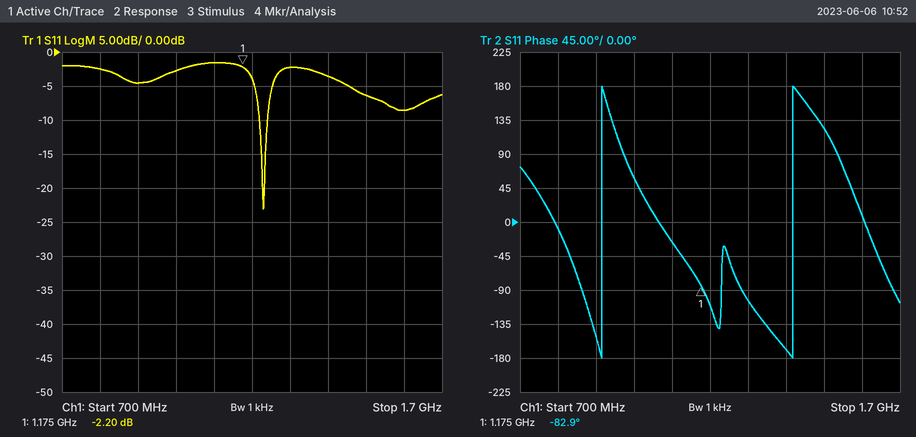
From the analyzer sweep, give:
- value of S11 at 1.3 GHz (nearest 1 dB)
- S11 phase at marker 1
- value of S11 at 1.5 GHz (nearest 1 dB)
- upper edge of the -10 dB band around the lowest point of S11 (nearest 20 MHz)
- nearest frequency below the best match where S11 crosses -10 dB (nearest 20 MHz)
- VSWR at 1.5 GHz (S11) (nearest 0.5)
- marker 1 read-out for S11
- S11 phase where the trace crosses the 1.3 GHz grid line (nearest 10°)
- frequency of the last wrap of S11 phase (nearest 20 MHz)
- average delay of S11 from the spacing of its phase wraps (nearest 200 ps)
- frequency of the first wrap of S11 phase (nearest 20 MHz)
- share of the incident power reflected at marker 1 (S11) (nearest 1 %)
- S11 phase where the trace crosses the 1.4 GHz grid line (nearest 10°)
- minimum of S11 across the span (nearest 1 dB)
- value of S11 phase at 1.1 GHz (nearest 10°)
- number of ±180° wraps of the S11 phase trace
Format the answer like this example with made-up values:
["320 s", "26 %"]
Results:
["-2 dB", "-82.9°", "-6 dB", "1.24 GHz", "1.22 GHz", "3.0", "-2.20 dB", "-100°", "1.42 GHz", "2.0 ns", "920 MHz", "60 %", "-170°", "-23 dB", "-30°", "2"]
